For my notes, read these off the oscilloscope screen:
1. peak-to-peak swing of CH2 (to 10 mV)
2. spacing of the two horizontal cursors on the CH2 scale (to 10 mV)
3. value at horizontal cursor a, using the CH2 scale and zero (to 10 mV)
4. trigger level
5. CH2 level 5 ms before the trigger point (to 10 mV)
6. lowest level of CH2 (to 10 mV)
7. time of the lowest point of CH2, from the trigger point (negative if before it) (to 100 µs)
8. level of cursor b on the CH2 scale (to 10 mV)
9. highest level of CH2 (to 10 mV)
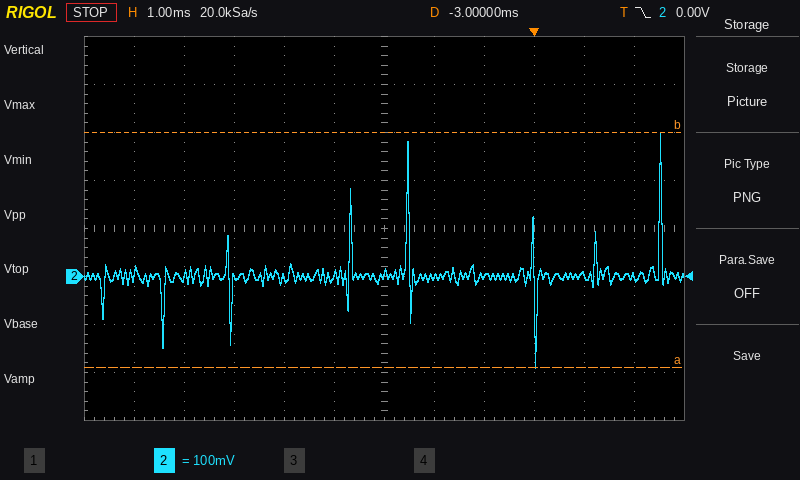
490 mV
490 mV
-190 mV
0.00 V
0 mV
-190 mV
0.0 ms
300 mV
300 mV
